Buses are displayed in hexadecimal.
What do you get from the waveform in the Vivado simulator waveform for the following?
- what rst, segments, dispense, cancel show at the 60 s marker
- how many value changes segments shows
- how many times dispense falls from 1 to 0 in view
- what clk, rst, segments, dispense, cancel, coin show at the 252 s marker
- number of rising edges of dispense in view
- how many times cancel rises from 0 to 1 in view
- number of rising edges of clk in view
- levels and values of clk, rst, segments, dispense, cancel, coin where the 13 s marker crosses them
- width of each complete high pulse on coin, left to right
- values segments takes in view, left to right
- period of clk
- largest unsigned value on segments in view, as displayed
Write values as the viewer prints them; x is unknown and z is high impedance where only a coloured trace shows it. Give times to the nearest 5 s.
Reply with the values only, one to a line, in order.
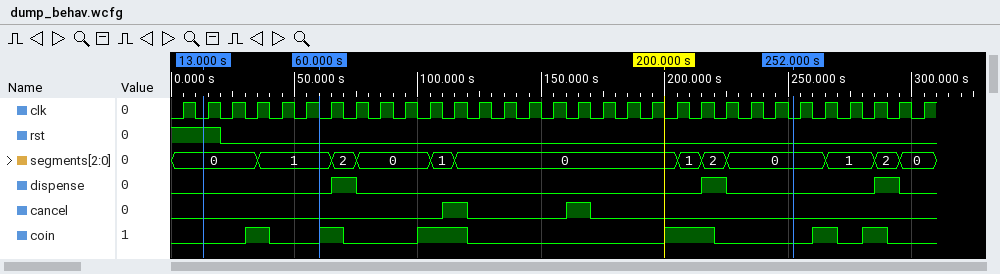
rst=0, segments=1, dispense=0, cancel=0
11
3
clk=0, rst=0, segments=0, dispense=0, cancel=0, coin=0
3
2
31
clk=0, rst=1, segments=0, dispense=0, cancel=0, coin=0
10 s, 10 s, 20 s, 20 s, 10 s, 10 s
0, 1, 2, 0, 1, 0, 1, 2, 0, 1, 2, 0
10 s
2
